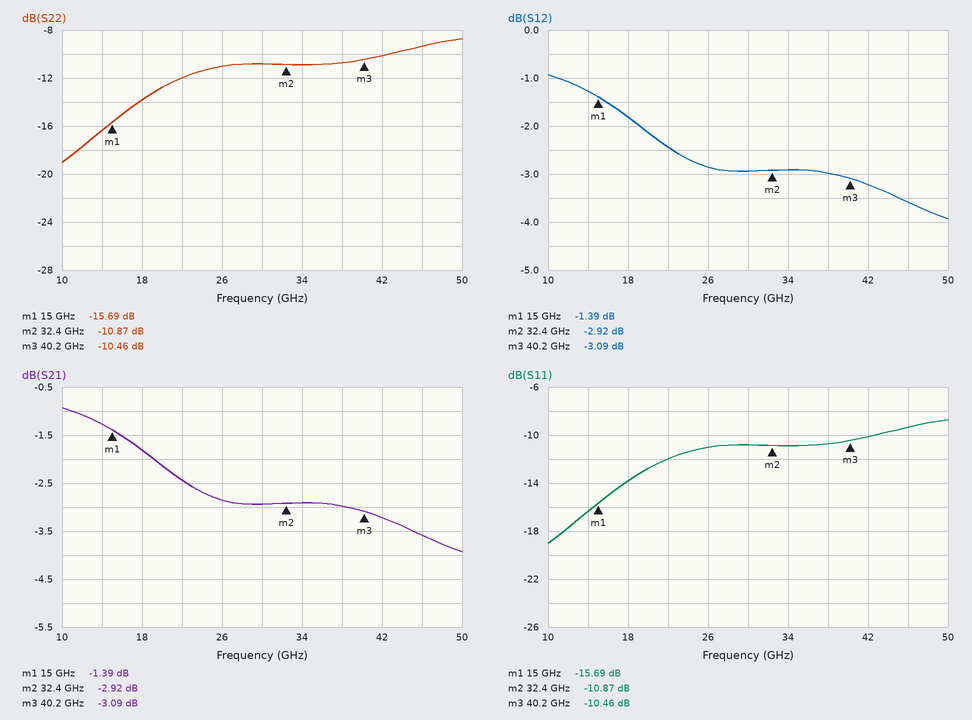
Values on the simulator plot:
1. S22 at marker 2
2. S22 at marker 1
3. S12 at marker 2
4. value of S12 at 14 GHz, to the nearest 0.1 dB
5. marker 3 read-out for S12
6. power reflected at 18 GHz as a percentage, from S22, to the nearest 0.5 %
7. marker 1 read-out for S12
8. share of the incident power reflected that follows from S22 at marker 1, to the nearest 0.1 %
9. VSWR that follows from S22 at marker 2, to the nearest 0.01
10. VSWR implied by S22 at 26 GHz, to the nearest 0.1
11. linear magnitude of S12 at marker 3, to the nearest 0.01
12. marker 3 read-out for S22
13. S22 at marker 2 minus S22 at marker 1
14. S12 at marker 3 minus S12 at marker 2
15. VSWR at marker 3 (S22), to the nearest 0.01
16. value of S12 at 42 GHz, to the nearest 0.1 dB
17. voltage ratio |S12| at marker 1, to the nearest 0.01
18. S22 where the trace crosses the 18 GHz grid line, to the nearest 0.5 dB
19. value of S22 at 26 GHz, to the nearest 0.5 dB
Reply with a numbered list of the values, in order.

1. -10.87 dB
2. -15.69 dB
3. -2.92 dB
4. -1.3 dB
5. -3.09 dB
6. 4.0 %
7. -1.39 dB
8. 2.7 %
9. 1.80
10. 1.8
11. 0.70
12. -10.46 dB
13. 4.82 dB
14. -0.17 dB
15. 1.86
16. -3.2 dB
17. 0.85
18. -14.0 dB
19. -11.0 dB
